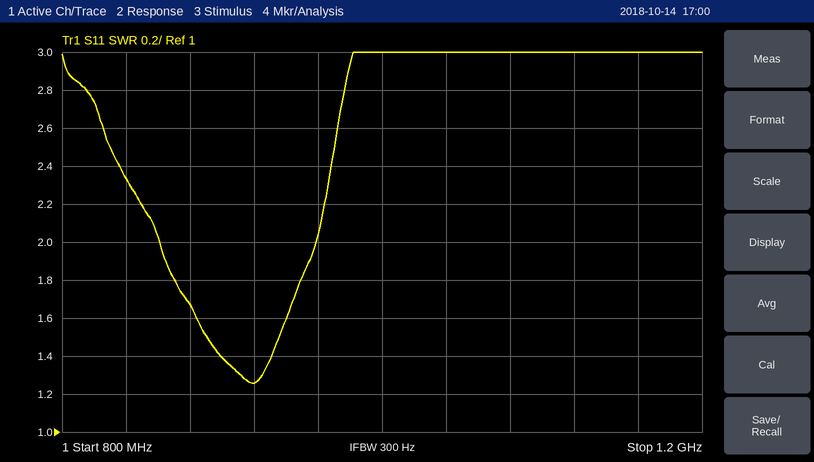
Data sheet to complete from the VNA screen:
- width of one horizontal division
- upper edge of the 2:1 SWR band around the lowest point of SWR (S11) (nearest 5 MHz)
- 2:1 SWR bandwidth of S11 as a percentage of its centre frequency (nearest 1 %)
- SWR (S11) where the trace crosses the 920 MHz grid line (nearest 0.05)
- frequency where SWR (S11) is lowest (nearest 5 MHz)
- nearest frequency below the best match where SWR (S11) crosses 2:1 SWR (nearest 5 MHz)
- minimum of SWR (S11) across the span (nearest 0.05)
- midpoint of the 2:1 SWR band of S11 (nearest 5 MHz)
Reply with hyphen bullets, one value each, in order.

- 40 MHz
- 960 MHz
- 11 %
- 1.25
- 920 MHz
- 860 MHz
- 1.25
- 910 MHz
